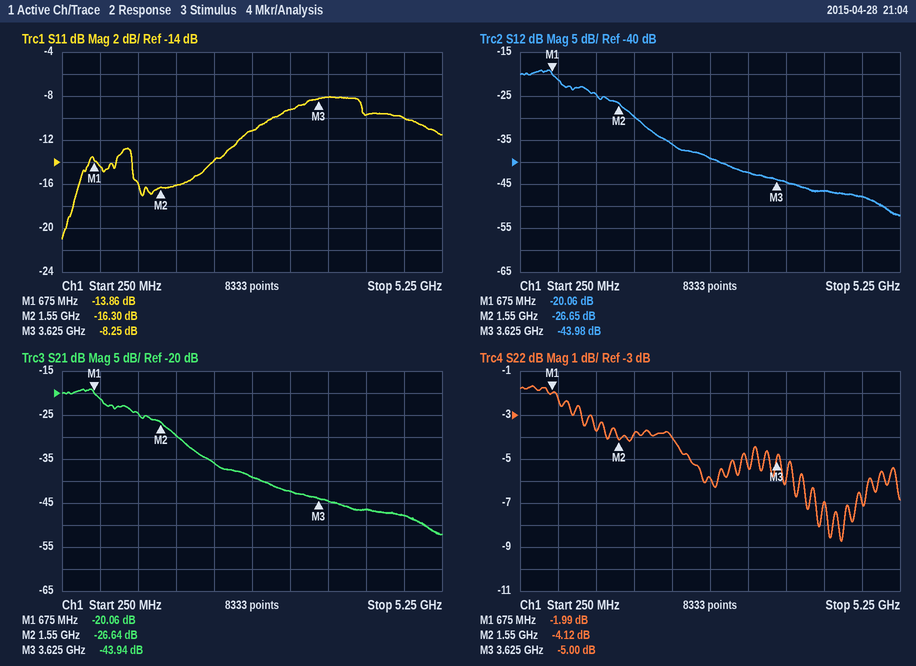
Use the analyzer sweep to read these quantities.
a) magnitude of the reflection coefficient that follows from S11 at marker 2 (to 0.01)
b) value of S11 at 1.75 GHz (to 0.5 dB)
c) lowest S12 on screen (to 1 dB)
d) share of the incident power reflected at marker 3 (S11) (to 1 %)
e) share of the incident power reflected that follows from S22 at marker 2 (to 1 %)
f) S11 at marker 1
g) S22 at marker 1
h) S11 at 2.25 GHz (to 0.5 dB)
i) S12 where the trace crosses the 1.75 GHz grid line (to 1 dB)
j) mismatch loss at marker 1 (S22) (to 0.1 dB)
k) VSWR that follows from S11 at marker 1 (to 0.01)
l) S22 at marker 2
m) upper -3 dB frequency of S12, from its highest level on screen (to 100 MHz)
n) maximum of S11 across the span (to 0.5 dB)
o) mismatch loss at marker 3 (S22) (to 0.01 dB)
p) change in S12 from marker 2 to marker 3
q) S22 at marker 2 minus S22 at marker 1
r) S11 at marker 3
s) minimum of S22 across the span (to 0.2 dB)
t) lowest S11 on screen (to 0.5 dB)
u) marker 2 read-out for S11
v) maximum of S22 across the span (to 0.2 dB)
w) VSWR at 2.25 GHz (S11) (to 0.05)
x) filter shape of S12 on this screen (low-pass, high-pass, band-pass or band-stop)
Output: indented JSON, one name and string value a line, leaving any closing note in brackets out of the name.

{
  "magnitude of the reflection coefficient that follows from S11 at marker 2": "0.15",
  "value of S11 at 1.75 GHz": "-16.0 dB",
  "lowest S12 on screen": "-52 dB",
  "share of the incident power reflected at marker 3 (S11)": "15 %",
  "share of the incident power reflected that follows from S22 at marker 2": "39 %",
  "S11 at marker 1": "-13.86 dB",
  "S22 at marker 1": "-1.99 dB",
  "S11 at 2.25 GHz": "-14.0 dB",
  "S12 where the trace crosses the 1.75 GHz grid line": "-30 dB",
  "mismatch loss at marker 1 (S22)": "4.3 dB",
  "VSWR that follows from S11 at marker 1": "1.51",
  "S22 at marker 2": "-4.12 dB",
  "upper -3 dB frequency of S12, from its highest level on screen": "800 MHz",
  "maximum of S11 across the span": "-8.0 dB",
  "mismatch loss at marker 3 (S22)": "1.65 dB",
  "change in S12 from marker 2 to marker 3": "-17.33 dB",
  "S22 at marker 2 minus S22 at marker 1": "-2.13 dB",
  "S11 at marker 3": "-8.25 dB",
  "minimum of S22 across the span": "-8.8 dB",
  "lowest S11 on screen": "-21.0 dB",
  "marker 2 read-out for S11": "-16.30 dB",
  "maximum of S22 across the span": "-1.6 dB",
  "VSWR at 2.25 GHz (S11)": "1.50",
  "filter shape of S12 on this screen": "low-pass"
}
